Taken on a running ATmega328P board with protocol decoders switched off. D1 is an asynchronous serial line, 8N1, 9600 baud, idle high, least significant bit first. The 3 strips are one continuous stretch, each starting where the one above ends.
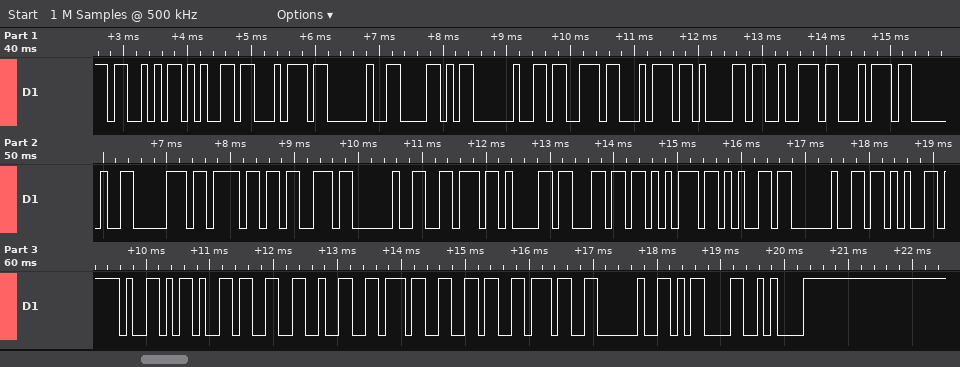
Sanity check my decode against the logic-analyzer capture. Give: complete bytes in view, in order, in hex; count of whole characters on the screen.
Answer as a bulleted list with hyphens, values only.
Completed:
- 53 65 74 20 58 20 73 74 61 72 74 20 70 6F 73 20 76 61 6C 75 65 20 2B 2F 2D 33 32 37 36 37 20 0D 0A
- 33
